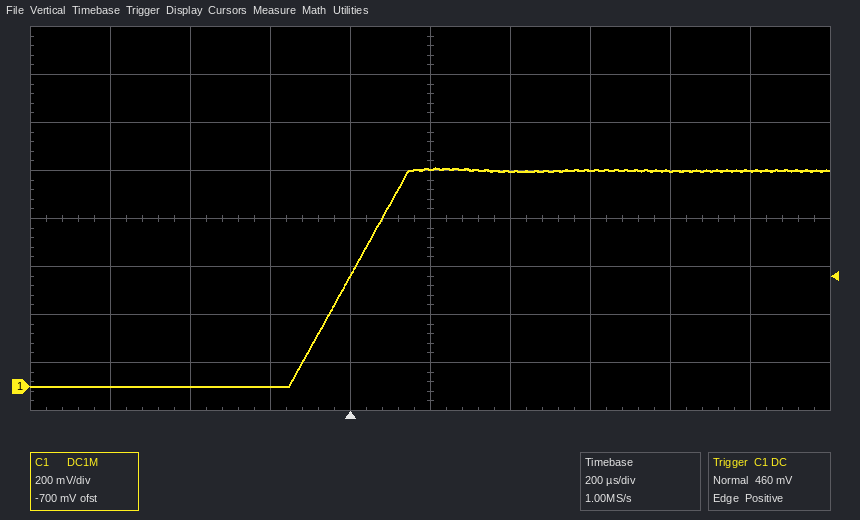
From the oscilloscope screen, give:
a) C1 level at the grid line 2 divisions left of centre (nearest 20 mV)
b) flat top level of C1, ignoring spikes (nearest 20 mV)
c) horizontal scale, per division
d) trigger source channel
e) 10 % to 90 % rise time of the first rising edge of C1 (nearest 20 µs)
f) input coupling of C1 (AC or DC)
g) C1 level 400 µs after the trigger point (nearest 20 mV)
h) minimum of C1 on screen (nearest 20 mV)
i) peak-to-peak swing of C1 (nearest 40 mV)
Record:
0 mV
900 mV
200 µs
C1
240 µs
DC
900 mV
0 mV
920 mV
